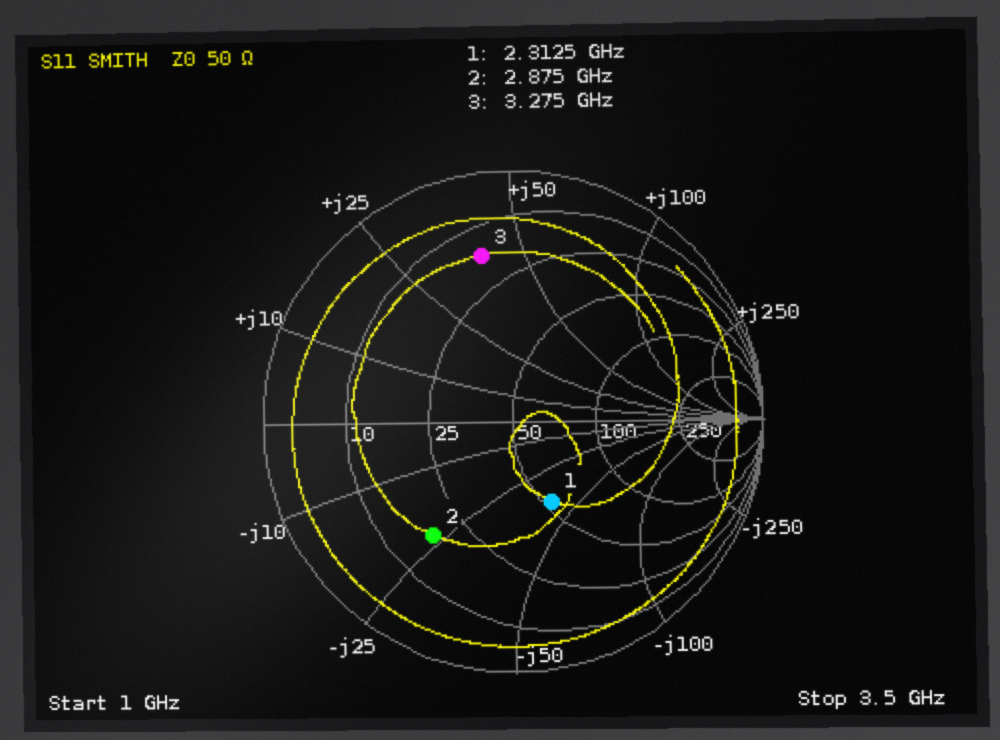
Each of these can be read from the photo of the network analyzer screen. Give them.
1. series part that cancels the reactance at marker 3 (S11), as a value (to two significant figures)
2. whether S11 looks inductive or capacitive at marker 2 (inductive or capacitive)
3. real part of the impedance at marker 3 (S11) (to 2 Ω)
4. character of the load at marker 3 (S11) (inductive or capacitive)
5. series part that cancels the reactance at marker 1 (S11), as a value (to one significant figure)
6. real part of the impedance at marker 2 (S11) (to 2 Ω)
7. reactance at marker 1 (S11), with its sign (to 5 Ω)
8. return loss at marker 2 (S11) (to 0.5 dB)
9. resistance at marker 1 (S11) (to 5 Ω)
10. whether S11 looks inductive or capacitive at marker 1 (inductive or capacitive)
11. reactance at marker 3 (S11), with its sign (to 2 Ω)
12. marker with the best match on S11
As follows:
1.2 pF
capacitive
16 Ω
inductive
3 nH
18 Ω
-40 Ω
5.0 dB
55 Ω
capacitive
+40 Ω
marker 1
